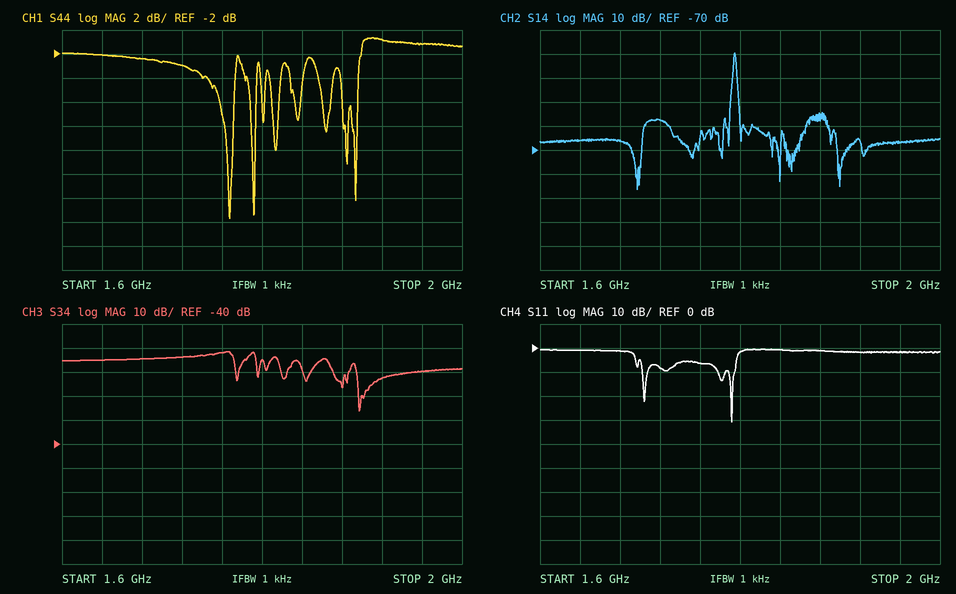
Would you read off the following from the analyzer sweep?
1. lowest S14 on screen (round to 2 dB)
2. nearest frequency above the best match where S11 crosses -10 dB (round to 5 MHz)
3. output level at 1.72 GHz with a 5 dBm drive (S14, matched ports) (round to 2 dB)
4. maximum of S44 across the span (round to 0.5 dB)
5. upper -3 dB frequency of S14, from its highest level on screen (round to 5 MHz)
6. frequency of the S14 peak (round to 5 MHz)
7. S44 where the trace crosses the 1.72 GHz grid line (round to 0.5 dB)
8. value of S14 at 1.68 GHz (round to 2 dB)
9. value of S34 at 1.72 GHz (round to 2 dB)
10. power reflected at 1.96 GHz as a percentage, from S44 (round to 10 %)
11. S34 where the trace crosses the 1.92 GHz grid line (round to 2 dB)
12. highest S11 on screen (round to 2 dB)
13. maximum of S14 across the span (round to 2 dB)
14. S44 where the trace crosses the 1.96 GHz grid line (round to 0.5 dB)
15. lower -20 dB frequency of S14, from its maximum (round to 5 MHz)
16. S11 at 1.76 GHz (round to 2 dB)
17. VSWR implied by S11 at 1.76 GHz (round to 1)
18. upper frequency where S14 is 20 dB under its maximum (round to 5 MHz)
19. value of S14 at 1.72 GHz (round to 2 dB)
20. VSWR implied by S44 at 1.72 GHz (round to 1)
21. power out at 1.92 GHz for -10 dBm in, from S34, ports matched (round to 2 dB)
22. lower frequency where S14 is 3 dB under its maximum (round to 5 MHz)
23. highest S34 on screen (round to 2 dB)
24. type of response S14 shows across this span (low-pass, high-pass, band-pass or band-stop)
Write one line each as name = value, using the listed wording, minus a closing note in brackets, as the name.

lowest S14 on screen = -86 dB
nearest frequency above the best match where S11 crosses -10 dB = 1.795 GHz
output level at 1.72 GHz with a 5 dBm drive (S14, matched ports) = -52 dBm
maximum of S44 across the span = -0.5 dB
upper -3 dB frequency of S14, from its highest level on screen = 1.795 GHz
frequency of the S14 peak = 1.795 GHz
S44 where the trace crosses the 1.72 GHz grid line = -3.0 dB
value of S14 at 1.68 GHz = -66 dB
value of S34 at 1.72 GHz = -4 dB
power reflected at 1.96 GHz as a percentage, from S44 = 80 %
S34 where the trace crosses the 1.92 GHz grid line = -12 dB
highest S11 on screen = 0 dB
maximum of S14 across the span = -30 dB
S44 where the trace crosses the 1.96 GHz grid line = -1.0 dB
lower -20 dB frequency of S14, from its maximum = 1.790 GHz
S11 at 1.76 GHz = -6 dB
VSWR implied by S11 at 1.76 GHz = 3
upper frequency where S14 is 20 dB under its maximum = 1.800 GHz
value of S14 at 1.72 GHz = -58 dB
VSWR implied by S44 at 1.72 GHz = 6
power out at 1.92 GHz for -10 dBm in, from S34, ports matched = -22 dBm
lower frequency where S14 is 3 dB under its maximum = 1.795 GHz
highest S34 on screen = -2 dB
type of response S14 shows across this span = band-pass
